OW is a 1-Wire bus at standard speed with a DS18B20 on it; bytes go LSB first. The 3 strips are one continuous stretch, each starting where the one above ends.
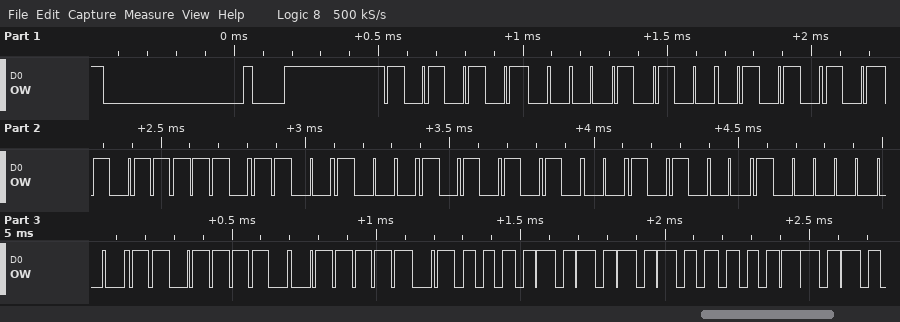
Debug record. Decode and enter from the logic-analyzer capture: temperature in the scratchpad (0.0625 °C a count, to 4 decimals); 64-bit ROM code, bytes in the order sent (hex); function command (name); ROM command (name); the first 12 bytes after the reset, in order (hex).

85.0000 °C
28 AA 7D 13 55 14 01 7B
Read Scratchpad
Match ROM
55 28 AA 7D 13 55 14 01 7B BE 50 05
